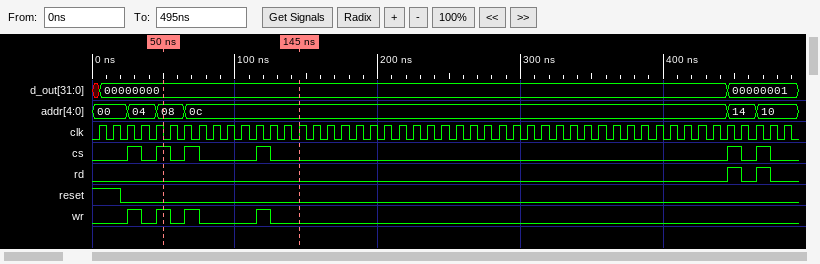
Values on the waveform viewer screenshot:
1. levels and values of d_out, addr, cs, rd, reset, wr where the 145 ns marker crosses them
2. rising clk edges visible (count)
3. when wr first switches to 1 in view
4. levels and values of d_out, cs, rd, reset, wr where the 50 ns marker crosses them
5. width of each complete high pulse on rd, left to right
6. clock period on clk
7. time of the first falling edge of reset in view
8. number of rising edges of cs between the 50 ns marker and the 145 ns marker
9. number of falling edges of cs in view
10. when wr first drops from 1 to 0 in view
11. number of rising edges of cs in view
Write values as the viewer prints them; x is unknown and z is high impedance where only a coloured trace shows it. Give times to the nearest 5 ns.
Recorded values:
d_out=00000000, addr=0c, cs=0, rd=0, reset=0, wr=0
49
25 ns
d_out=00000000, cs=1, rd=0, reset=0, wr=1
10 ns, 10 ns
10 ns
20 ns
2
6
35 ns
6
